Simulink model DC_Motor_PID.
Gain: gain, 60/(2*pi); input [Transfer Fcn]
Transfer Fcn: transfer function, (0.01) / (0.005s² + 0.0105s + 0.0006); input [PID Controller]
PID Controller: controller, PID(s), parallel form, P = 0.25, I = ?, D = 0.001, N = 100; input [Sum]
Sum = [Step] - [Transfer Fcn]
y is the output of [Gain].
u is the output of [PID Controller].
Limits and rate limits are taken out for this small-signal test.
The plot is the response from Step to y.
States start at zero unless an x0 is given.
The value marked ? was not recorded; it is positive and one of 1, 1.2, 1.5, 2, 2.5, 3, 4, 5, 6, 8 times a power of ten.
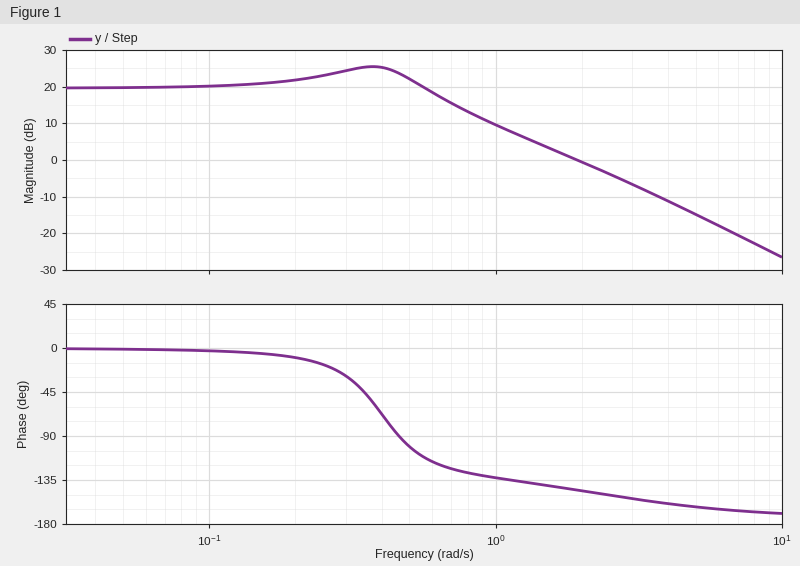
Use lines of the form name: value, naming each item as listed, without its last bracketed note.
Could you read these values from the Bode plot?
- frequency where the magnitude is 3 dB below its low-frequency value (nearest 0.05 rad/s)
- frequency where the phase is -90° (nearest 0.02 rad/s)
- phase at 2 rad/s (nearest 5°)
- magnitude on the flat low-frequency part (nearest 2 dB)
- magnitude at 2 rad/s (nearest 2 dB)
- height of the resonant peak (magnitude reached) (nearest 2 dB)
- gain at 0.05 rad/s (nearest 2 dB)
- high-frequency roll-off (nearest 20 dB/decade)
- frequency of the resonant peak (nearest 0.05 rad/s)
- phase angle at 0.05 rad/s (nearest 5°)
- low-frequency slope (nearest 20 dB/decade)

frequency where the magnitude is 3 dB below its low-frequency value: 0.65 rad/s
frequency where the phase is -90°: 0.46 rad/s
phase at 2 rad/s: -145°
magnitude on the flat low-frequency part: 20 dB
magnitude at 2 rad/s: 0 dB
height of the resonant peak (magnitude reached): 26 dB
gain at 0.05 rad/s: 20 dB
high-frequency roll-off: -40 dB/decade
frequency of the resonant peak: 0.35 rad/s
phase angle at 0.05 rad/s: 0°
low-frequency slope: 0 dB/decade
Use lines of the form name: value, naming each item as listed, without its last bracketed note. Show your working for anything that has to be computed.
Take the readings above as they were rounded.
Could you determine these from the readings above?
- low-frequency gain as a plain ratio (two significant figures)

low-frequency gain as a plain ratio: 10^(20 / 20) = 10
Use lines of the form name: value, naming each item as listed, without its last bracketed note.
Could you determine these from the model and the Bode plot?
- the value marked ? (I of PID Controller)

the value marked ?: 0.15
